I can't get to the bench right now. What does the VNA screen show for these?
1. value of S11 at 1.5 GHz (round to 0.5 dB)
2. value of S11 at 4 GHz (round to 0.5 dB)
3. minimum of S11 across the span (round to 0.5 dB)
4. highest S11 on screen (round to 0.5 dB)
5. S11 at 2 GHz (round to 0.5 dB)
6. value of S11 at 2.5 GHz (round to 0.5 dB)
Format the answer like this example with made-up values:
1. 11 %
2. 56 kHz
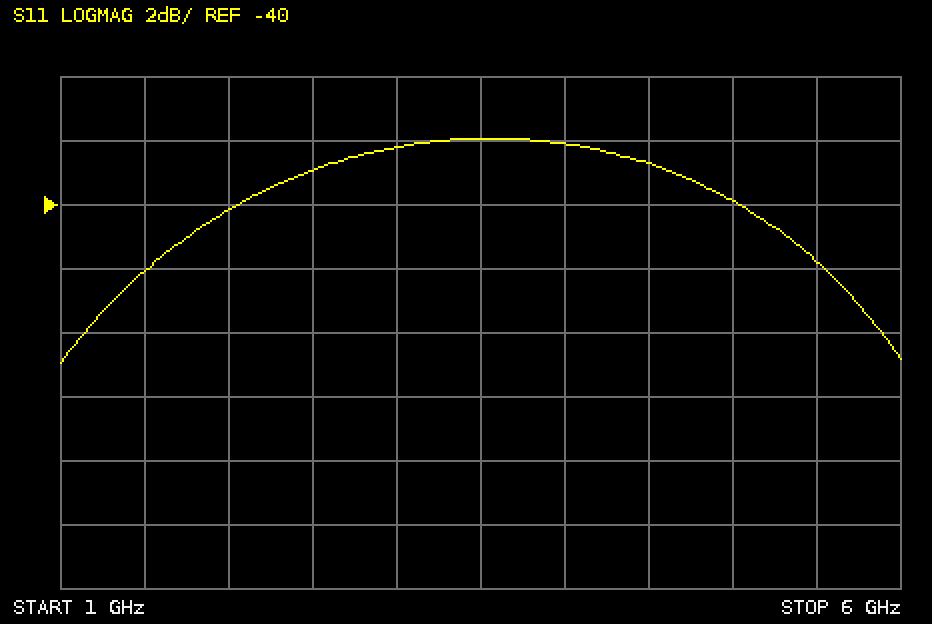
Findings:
1. -42.0 dB
2. -38.0 dB
3. -45.0 dB
4. -38.0 dB
5. -40.0 dB
6. -39.0 dB
